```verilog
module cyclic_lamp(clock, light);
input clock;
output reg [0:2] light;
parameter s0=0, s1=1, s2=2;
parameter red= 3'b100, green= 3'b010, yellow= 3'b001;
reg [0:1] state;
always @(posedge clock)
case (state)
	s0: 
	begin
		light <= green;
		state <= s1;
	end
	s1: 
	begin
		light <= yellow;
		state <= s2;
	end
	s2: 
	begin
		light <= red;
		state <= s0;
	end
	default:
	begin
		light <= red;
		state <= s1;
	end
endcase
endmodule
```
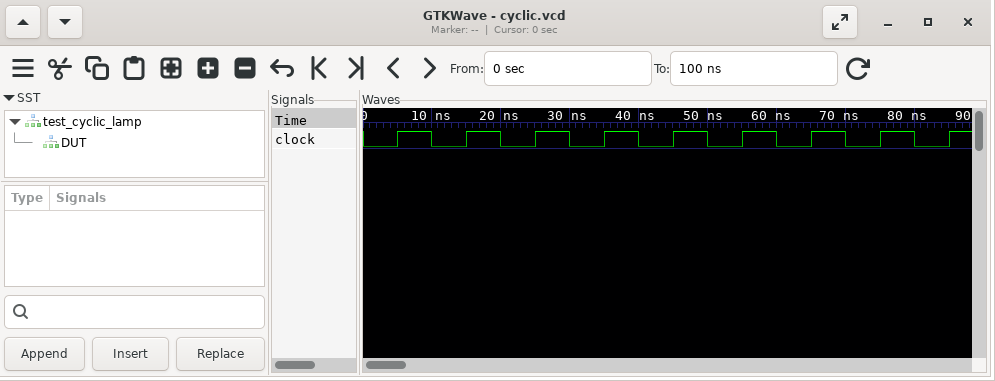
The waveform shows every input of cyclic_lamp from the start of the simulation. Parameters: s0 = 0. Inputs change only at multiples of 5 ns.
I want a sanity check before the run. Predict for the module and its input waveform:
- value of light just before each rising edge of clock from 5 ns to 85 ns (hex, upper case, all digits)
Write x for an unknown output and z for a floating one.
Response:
x, 4, 1, 4, 2, 1, 4, 2, 1
